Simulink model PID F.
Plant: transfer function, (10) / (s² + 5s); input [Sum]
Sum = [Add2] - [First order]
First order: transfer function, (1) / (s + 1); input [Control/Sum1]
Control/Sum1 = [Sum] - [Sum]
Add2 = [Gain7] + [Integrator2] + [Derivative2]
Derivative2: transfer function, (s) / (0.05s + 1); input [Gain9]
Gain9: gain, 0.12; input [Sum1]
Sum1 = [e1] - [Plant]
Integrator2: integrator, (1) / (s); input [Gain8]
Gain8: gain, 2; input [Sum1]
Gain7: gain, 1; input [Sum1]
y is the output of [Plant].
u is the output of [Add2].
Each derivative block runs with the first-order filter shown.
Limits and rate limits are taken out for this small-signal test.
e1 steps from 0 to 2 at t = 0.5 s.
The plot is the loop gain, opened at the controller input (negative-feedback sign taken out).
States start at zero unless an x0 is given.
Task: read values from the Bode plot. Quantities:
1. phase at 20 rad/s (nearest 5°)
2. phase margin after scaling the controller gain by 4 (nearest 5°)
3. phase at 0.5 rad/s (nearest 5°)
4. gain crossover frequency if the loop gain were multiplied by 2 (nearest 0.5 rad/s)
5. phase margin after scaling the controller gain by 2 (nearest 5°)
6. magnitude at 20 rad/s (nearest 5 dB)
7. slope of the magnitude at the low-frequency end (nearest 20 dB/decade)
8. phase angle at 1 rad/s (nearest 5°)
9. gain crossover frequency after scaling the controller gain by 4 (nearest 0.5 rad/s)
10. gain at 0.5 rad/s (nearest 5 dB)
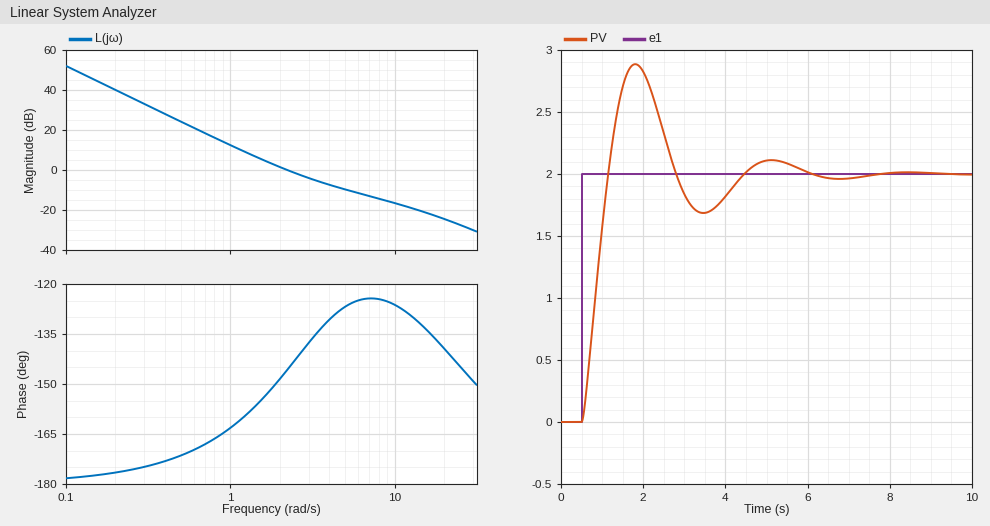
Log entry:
-140°
55°
-170°
3.5 rad/s
45°
-25 dB
-40 dB/decade
-165°
6.5 rad/s
25 dB
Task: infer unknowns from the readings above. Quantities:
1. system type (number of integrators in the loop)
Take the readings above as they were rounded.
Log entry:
2
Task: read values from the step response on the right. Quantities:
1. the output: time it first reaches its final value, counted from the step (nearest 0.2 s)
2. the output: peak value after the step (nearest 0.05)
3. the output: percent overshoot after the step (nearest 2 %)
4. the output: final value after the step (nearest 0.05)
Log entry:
0.6 s
2.90
44 %
2.00
